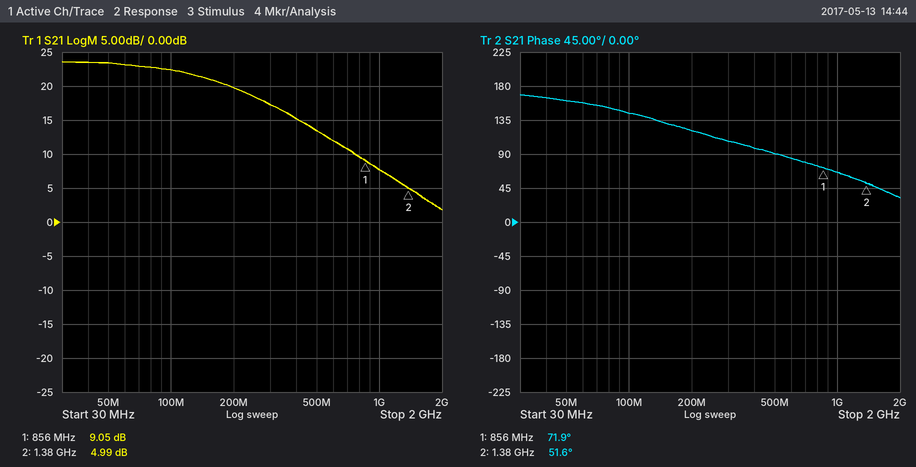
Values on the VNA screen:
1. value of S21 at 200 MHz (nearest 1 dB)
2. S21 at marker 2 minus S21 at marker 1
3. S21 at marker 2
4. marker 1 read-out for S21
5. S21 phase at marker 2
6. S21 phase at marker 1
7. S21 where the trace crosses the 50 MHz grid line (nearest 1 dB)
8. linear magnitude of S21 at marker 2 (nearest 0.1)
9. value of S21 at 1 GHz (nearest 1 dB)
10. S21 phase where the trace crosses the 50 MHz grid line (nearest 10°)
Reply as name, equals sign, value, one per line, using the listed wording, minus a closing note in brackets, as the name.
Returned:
value of S21 at 200 MHz = 20 dB
S21 at marker 2 minus S21 at marker 1 = -4.06 dB
S21 at marker 2 = 4.99 dB
marker 1 read-out for S21 = 9.05 dB
S21 phase at marker 2 = 51.6°
S21 phase at marker 1 = 71.9°
S21 where the trace crosses the 50 MHz grid line = 23 dB
linear magnitude of S21 at marker 2 = 1.8
value of S21 at 1 GHz = 8 dB
S21 phase where the trace crosses the 50 MHz grid line = 160°
